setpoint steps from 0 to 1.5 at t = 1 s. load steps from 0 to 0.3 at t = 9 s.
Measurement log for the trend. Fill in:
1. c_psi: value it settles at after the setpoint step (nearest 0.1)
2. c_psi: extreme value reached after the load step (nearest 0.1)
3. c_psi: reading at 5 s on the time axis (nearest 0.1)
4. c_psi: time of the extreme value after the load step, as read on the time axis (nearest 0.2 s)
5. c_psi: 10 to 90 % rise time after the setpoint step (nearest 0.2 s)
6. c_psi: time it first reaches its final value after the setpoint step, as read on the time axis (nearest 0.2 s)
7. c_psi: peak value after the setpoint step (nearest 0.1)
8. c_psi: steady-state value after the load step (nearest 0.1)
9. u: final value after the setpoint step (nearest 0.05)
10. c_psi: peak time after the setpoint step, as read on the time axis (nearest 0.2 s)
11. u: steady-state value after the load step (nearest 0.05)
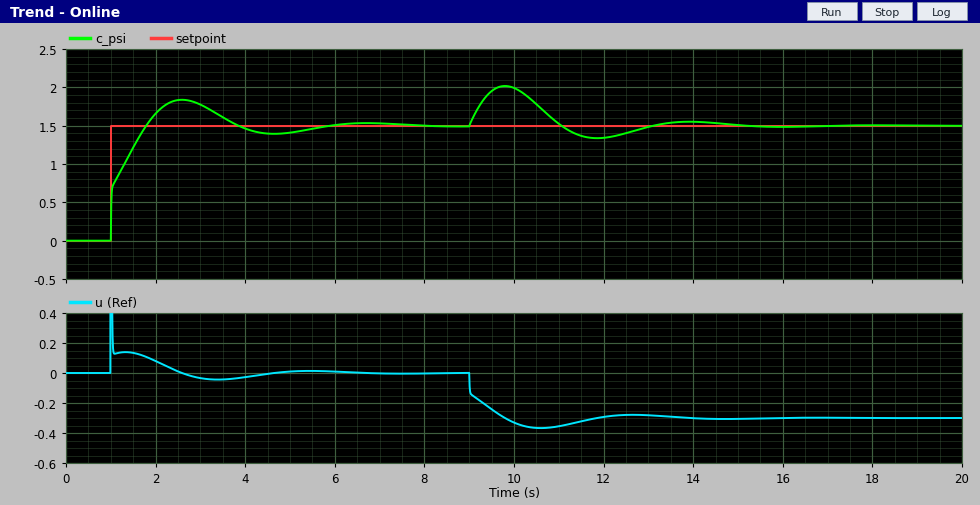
1.5
2.0
1.4
9.8 s
0.6 s
1.8 s
1.8
1.5
0.00
2.6 s
-0.30
